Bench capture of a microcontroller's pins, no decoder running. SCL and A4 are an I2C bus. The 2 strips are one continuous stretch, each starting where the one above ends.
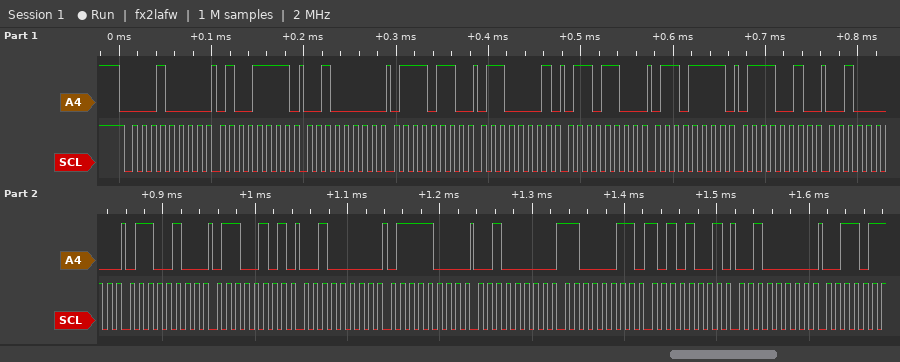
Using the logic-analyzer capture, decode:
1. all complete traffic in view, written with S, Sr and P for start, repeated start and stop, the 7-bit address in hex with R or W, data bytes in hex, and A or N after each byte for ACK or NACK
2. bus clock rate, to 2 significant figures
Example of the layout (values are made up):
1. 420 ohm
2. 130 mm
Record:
1. S 08W A 4F A 20 A 76 A 61 A 6C A 6F A 72 A 20 A 64 A 65 A 20 A 78 A 20 A C3 A A9 A 20 A
2. 100 kHz
